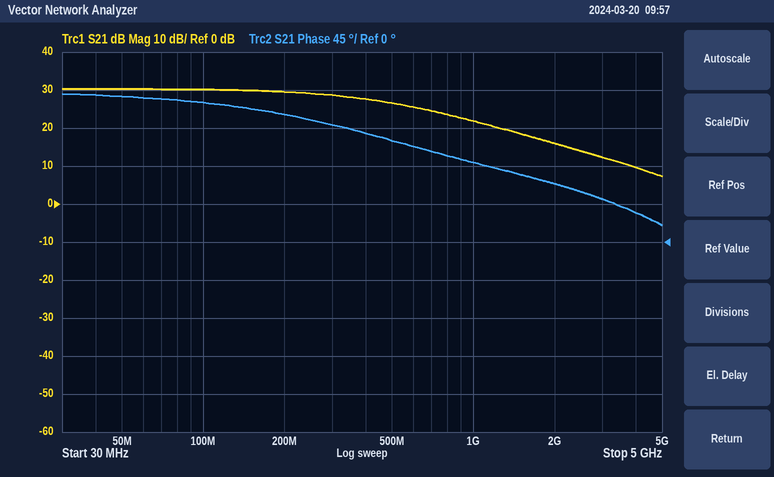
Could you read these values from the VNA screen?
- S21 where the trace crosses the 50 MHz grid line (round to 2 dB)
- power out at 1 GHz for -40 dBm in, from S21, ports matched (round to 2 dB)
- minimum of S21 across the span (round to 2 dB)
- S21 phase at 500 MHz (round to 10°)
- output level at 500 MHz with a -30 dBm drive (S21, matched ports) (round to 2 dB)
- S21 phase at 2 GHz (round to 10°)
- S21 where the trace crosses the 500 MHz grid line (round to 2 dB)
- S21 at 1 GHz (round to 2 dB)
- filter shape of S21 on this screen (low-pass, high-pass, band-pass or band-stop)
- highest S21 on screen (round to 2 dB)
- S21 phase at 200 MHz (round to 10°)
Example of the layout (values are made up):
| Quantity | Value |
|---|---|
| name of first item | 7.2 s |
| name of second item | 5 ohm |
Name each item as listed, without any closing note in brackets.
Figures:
| Quantity | Value |
|---|---|
| S21 where the trace crosses the 50 MHz grid line | 30 dB |
| power out at 1 GHz for -40 dBm in, from S21, ports matched | -18 dBm |
| minimum of S21 across the span | 8 dB |
| S21 phase at 500 MHz | 120° |
| output level at 500 MHz with a -30 dBm drive (S21, matched ports) | -4 dBm |
| S21 phase at 2 GHz | 70° |
| S21 where the trace crosses the 500 MHz grid line | 26 dB |
| S21 at 1 GHz | 22 dB |
| filter shape of S21 on this screen | low-pass |
| highest S21 on screen | 30 dB |
| S21 phase at 200 MHz | 150° |
